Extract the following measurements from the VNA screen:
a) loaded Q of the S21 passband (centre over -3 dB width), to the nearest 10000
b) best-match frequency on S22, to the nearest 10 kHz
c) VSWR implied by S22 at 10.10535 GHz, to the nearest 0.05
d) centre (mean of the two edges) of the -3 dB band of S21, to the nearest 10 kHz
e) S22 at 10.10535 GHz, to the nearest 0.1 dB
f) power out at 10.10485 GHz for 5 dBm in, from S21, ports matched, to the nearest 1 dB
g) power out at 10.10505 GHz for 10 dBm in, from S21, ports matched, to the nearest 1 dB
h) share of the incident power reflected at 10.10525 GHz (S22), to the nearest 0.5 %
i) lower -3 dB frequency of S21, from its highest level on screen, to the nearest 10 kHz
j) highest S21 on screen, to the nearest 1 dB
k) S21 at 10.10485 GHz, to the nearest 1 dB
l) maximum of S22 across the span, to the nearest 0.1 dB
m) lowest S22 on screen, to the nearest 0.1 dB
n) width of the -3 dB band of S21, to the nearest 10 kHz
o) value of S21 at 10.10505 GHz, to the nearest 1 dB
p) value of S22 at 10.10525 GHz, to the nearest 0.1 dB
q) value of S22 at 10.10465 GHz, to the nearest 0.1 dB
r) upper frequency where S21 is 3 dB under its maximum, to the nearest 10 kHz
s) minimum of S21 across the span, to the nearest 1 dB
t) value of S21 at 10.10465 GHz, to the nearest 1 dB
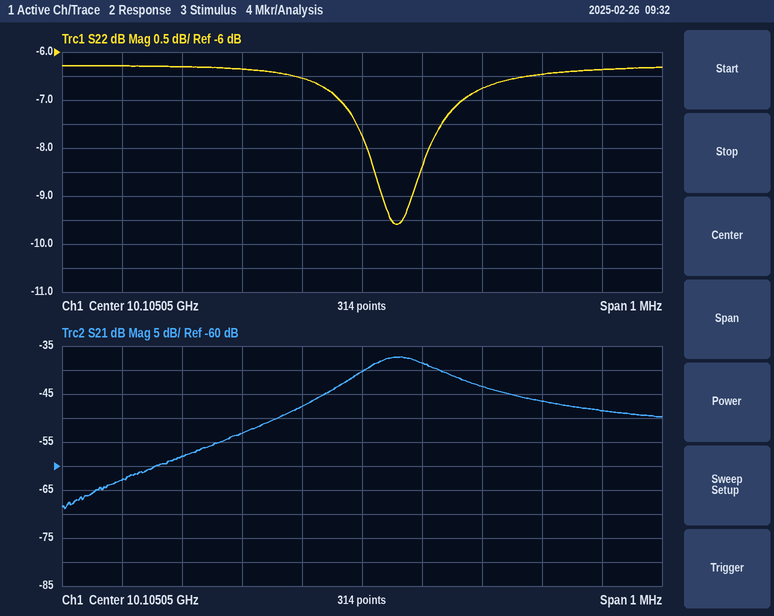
80000
10.10511 GHz
2.80
10.10512 GHz
-6.5 dB
-48 dBm
-30 dBm
21.0 %
10.10505 GHz
-37 dB
-53 dB
-6.3 dB
-9.6 dB
130 kHz
-40 dB
-6.8 dB
-6.3 dB
10.10518 GHz
-69 dB
-63 dB
